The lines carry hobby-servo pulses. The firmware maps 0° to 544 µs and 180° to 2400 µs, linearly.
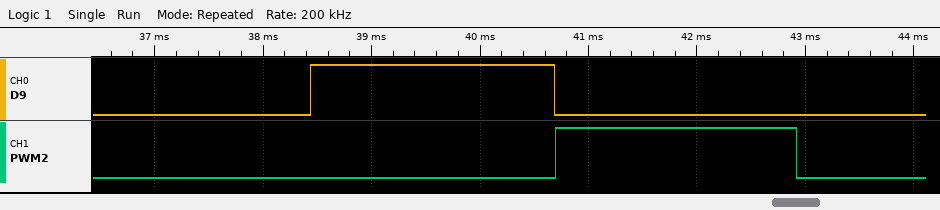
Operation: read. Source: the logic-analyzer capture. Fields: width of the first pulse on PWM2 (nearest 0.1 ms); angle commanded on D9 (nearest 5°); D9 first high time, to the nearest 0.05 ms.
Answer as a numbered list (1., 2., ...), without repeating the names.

1. 2.2 ms
2. 165°
3. 2.25 ms
